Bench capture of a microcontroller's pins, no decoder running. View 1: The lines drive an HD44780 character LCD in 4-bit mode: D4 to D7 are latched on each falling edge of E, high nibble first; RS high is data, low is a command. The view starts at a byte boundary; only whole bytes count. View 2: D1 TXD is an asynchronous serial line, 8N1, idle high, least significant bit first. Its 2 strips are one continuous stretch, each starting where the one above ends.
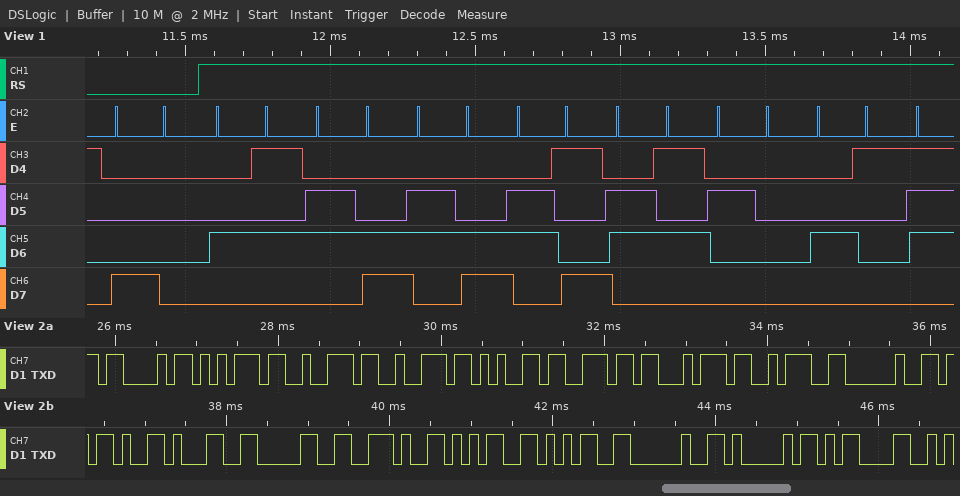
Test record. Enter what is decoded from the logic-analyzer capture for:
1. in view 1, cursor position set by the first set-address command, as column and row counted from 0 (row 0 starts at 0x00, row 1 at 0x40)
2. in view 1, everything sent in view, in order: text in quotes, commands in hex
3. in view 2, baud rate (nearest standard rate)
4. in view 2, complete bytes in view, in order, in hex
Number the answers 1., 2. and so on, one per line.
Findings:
1. column 0, row 0
2. 0x80 "Ellie A"
3. 9600 baud
4. 43 75 72 72 65 6E 74 3A 20 2D 31 30 2E 35 35 20 41 0D
